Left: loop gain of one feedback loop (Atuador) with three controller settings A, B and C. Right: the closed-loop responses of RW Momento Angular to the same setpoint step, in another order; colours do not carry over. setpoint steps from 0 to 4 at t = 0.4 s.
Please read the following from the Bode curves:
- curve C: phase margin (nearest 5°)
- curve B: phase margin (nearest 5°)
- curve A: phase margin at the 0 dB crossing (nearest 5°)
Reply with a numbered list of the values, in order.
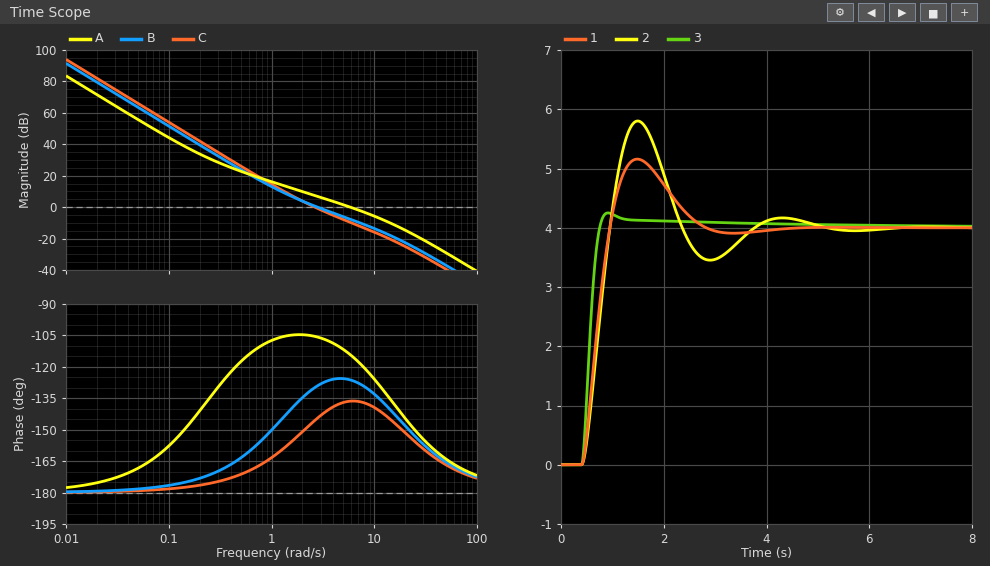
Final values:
1. 35°
2. 50°
3. 65°
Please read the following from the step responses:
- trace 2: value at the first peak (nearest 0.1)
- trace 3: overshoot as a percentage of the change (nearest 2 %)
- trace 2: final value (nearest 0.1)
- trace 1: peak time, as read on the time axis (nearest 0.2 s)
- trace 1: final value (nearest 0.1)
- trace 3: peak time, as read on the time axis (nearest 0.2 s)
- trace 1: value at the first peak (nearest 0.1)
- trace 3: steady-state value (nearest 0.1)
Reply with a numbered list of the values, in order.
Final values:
1. 5.8
2. 6 %
3. 4.0
4. 1.4 s
5. 4.0
6. 1.0 s
7. 5.2
8. 4.0
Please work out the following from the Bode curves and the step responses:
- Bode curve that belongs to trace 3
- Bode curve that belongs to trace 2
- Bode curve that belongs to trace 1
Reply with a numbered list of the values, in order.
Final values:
1. A
2. C
3. B
